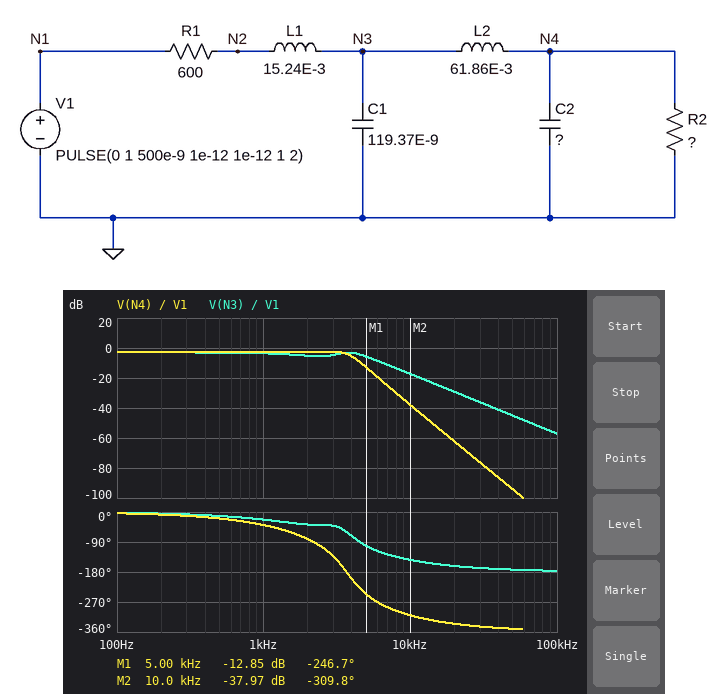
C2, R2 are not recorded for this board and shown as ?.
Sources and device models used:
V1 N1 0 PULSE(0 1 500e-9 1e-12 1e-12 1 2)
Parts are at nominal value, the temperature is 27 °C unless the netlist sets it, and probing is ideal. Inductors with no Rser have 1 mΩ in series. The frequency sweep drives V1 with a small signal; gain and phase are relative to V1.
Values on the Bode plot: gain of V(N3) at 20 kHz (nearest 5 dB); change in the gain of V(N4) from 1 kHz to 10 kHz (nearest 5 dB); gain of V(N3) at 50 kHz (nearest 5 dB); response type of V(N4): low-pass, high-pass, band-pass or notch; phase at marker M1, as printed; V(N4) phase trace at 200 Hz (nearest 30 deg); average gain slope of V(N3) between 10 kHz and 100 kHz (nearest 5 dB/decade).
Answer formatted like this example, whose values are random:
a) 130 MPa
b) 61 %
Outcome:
a) -30 dB
b) -35 dB
c) -45 dB
d) low-pass
e) -246.7 deg
f) 0 deg
g) -40 dB/decade
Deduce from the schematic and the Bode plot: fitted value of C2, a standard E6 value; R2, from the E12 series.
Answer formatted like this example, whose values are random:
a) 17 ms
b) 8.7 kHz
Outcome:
a) 47 nF
b) 1.5 kΩ
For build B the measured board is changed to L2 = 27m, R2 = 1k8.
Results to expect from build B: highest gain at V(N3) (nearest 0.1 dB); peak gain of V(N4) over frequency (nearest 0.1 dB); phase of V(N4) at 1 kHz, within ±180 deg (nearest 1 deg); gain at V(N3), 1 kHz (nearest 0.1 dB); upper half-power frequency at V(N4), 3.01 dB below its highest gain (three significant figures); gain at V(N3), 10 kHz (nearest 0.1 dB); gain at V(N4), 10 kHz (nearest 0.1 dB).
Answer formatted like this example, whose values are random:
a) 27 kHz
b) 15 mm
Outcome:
a) -2.5 dB
b) -1.9 dB
c) -33 deg
d) -3.1 dB
e) 5.89 kHz
f) -16.7 dB
g) -29.0 dB
